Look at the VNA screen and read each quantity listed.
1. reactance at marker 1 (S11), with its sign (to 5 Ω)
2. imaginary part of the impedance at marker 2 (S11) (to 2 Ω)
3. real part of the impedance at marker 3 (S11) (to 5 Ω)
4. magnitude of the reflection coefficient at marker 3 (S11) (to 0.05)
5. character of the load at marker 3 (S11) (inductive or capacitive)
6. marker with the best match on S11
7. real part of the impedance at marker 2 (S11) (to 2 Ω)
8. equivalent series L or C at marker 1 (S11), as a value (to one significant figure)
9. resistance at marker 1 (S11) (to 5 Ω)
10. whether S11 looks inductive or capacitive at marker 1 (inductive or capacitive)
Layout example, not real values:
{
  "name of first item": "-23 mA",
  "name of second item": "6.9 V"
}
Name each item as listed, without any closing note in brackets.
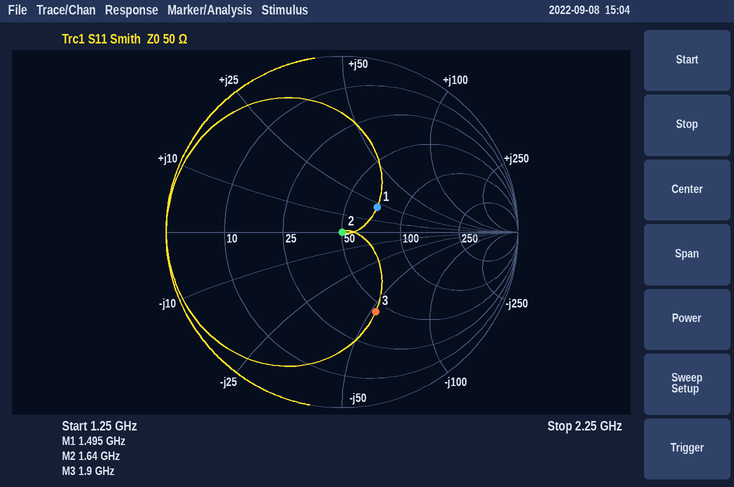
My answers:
{
  "reactance at marker 1 (S11), with its sign": "+20 Ω",
  "imaginary part of the impedance at marker 2 (S11)": "0 Ω",
  "real part of the impedance at marker 3 (S11)": "45 Ω",
  "magnitude of the reflection coefficient at marker 3 (S11)": "0.50",
  "character of the load at marker 3 (S11)": "capacitive",
  "marker with the best match on S11": "marker 2",
  "real part of the impedance at marker 2 (S11)": "50 Ω",
  "equivalent series L or C at marker 1 (S11), as a value": "2 nH",
  "resistance at marker 1 (S11)": "70 Ω",
  "whether S11 looks inductive or capacitive at marker 1": "inductive"
}
